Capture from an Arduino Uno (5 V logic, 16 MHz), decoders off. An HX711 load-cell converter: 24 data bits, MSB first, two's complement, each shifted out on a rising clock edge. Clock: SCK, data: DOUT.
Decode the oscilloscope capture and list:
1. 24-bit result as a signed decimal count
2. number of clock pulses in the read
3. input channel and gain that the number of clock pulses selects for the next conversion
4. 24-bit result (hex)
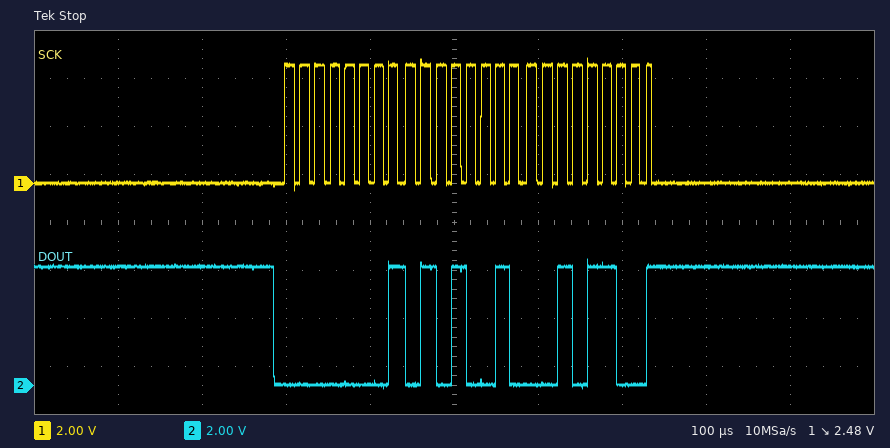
86572
25
channel A, gain 128
0x01522C
